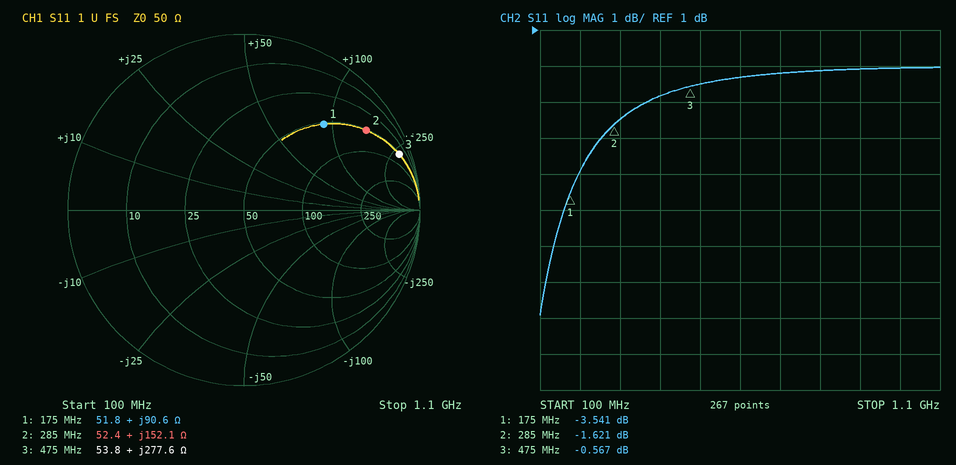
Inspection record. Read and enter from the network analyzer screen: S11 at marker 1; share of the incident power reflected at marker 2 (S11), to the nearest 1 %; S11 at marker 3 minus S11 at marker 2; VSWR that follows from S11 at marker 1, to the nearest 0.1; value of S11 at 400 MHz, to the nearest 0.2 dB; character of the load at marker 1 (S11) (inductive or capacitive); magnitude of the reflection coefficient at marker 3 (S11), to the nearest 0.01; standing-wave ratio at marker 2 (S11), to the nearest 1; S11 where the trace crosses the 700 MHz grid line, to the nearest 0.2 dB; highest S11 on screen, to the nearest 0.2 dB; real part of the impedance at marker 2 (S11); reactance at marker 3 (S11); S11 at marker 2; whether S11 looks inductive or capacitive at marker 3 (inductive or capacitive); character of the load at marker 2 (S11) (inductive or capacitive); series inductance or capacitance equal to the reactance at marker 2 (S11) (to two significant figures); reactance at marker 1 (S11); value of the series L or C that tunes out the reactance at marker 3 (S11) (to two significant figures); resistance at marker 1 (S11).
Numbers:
-3.541 dB
69 %
1.054 dB
5.0
-0.8 dB
inductive
0.94
11
-0.2 dB
0.0 dB
52.4 Ω
+277.6 Ω
-1.621 dB
inductive
inductive
85 nH
+90.6 Ω
1.2 pF
51.8 Ω
